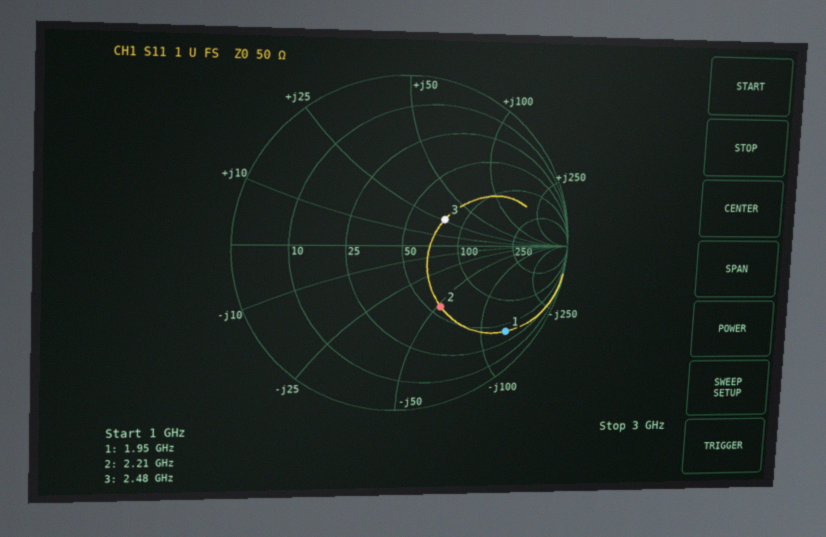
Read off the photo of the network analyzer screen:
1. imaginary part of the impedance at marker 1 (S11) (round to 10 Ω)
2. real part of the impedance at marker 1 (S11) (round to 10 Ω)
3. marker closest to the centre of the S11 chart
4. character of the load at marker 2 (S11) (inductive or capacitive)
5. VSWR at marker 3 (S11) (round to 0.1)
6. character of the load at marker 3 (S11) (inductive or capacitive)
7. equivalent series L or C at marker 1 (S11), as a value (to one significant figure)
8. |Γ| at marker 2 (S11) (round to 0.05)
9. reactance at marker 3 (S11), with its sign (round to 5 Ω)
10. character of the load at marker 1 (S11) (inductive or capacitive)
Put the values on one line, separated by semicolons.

-130 Ω; 40 Ω; marker 3; capacitive; 1.8; inductive; 600 fF; 0.45; +25 Ω; capacitive
